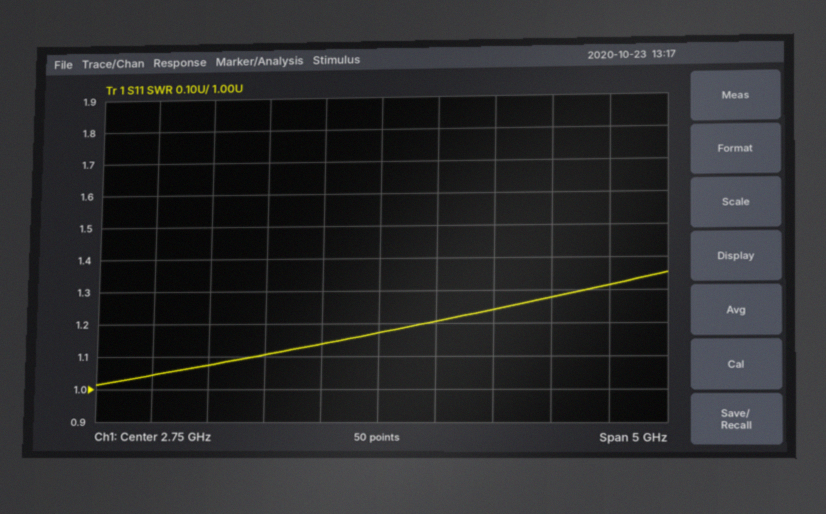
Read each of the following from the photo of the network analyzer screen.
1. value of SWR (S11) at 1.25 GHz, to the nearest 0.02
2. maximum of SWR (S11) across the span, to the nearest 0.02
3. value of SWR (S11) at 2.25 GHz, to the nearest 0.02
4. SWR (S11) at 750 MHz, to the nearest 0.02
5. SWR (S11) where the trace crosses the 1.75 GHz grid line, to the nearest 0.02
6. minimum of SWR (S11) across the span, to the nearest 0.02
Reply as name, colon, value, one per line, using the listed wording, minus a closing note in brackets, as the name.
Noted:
value of SWR (S11) at 1.25 GHz, to the nearest 0.02: 1.08
maximum of SWR (S11) across the span, to the nearest 0.02: 1.36
value of SWR (S11) at 2.25 GHz, to the nearest 0.02: 1.14
SWR (S11) at 750 MHz, to the nearest 0.02: 1.04
SWR (S11) where the trace crosses the 1.75 GHz grid line, to the nearest 0.02: 1.10
minimum of SWR (S11) across the span, to the nearest 0.02: 1.02
